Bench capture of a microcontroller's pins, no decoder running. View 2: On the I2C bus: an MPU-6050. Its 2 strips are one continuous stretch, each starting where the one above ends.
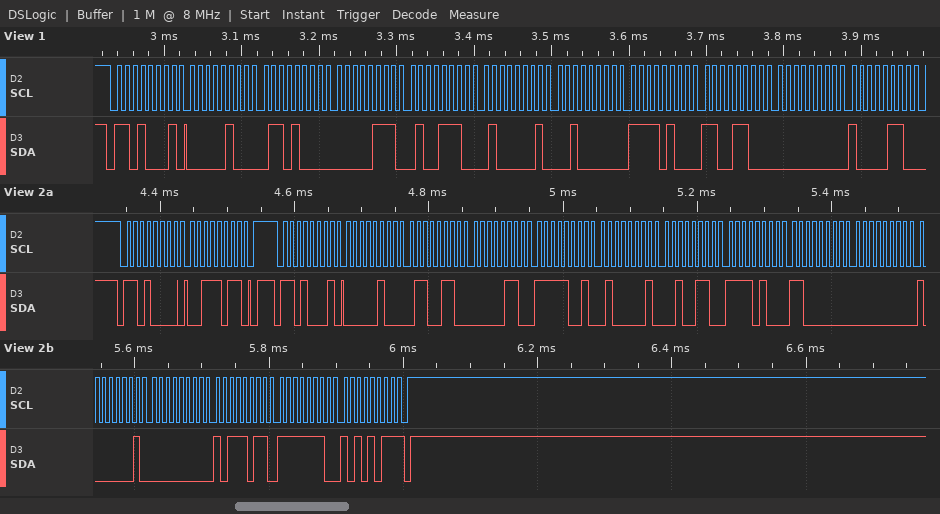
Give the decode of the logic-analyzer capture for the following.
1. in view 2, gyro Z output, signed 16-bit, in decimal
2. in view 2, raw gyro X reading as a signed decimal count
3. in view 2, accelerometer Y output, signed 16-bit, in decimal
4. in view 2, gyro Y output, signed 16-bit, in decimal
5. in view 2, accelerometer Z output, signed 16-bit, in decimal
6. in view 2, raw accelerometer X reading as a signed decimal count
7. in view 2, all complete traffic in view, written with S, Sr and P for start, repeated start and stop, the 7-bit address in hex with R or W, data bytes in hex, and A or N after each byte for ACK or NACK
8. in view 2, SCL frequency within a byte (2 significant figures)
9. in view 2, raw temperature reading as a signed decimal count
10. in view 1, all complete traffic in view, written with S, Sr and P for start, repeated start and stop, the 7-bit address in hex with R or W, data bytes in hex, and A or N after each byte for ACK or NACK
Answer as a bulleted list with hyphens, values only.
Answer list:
- -341
- 129
- 1785
- 187
- 16678
- 1126
- S 68W A 3B A P S 68R A 04 A 66 A 06 A F9 A 41 A 26 A F4 A C0 A 00 A 81 A 00 A BB A FE A AB N P
- 100 kHz
- -2880
- S 68R A 04 A 68 A 07 A 4E A 41 A 20 A F4 A CC A 00 A 86 A
